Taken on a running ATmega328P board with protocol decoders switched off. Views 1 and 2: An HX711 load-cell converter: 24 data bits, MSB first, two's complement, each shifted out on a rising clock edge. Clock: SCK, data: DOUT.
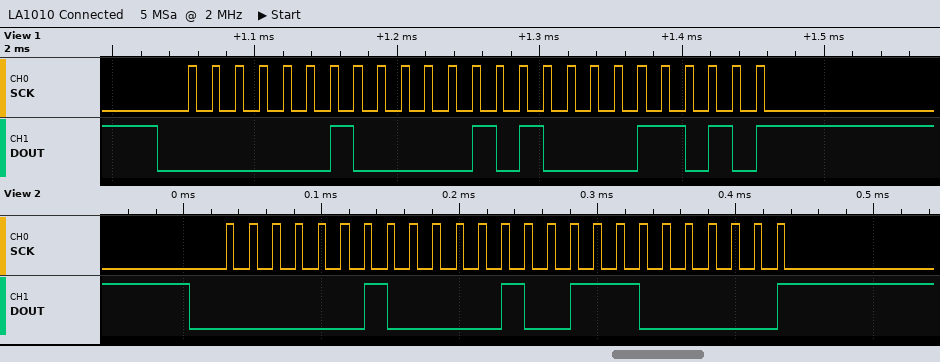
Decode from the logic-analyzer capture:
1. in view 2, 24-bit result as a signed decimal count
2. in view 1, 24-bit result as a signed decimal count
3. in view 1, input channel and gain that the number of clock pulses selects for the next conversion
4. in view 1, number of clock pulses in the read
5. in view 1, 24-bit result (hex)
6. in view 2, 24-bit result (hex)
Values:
133568
133658
channel A, gain 128
25
0x020A1A
0x0209C0
